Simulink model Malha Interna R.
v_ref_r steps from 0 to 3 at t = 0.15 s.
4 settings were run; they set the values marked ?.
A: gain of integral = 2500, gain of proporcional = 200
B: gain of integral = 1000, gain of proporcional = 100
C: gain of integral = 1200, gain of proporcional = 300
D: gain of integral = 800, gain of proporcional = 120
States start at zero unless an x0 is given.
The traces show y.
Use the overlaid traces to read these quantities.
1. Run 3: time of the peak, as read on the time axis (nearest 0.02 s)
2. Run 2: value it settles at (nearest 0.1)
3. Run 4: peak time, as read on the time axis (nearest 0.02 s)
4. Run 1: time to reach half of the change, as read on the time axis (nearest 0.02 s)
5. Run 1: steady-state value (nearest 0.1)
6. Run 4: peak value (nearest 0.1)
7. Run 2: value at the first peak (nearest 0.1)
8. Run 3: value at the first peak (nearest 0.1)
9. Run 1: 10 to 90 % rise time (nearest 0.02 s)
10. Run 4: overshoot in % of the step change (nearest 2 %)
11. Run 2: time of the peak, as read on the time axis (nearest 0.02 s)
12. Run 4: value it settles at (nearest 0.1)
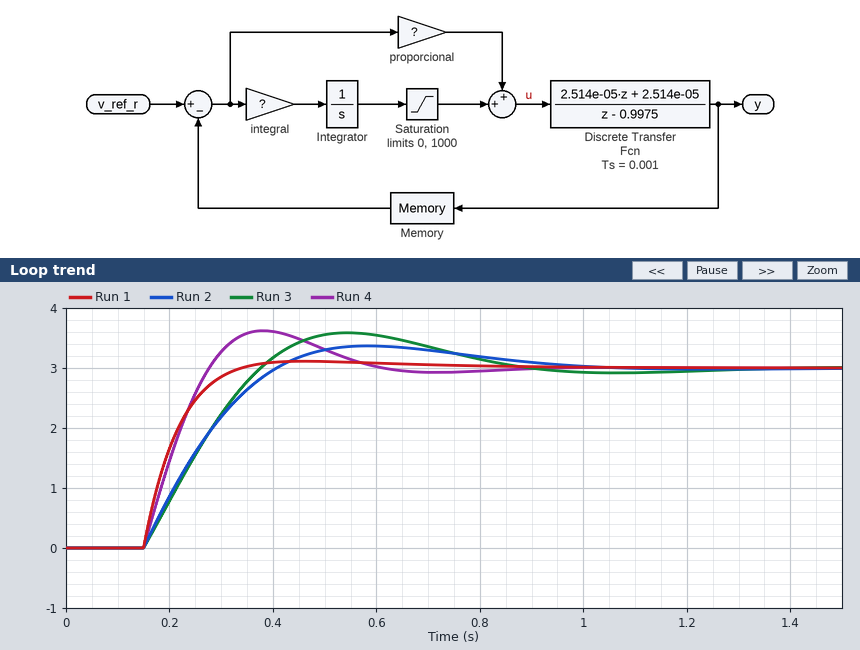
0.54 s
3.0
0.38 s
0.20 s
3.0
3.6
3.4
3.6
0.12 s
20 %
0.58 s
3.0
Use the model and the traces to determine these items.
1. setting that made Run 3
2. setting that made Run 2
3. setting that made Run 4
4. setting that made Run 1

B
D
A
C
